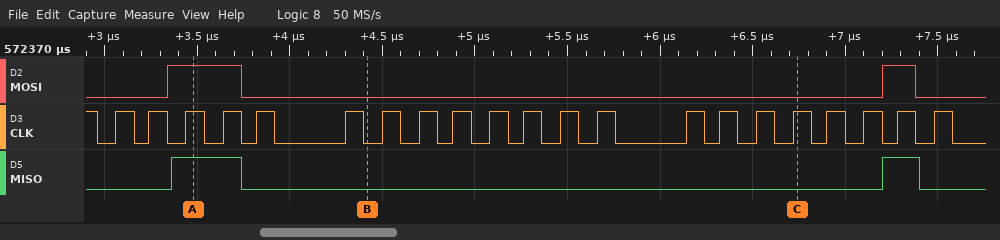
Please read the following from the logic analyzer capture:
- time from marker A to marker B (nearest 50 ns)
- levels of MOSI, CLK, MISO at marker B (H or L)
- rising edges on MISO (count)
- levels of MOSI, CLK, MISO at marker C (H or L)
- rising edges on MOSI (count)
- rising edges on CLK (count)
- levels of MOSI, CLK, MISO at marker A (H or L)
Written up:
950 ns
MOSI=L, CLK=L, MISO=L
2
MOSI=L, CLK=H, MISO=L
2
21
MOSI=H, CLK=H, MISO=H
